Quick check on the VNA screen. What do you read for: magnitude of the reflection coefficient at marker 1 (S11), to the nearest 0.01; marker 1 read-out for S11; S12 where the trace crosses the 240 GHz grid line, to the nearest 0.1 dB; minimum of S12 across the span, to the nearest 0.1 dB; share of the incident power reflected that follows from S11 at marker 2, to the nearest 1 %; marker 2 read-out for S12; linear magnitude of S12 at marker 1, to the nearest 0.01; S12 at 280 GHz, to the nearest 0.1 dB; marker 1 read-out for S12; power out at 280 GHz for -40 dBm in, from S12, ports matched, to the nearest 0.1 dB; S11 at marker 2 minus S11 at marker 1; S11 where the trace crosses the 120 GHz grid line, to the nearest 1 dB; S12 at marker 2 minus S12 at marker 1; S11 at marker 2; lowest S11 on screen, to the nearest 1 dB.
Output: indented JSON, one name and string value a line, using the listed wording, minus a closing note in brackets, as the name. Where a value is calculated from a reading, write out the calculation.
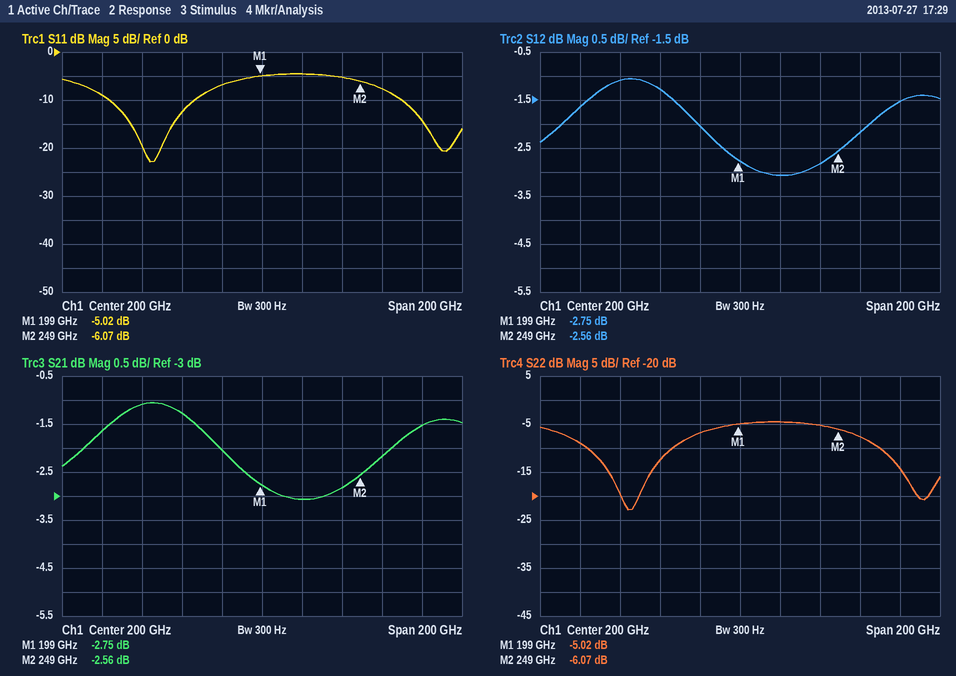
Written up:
{
  "magnitude of the reflection coefficient at marker 1 (S11), to the nearest 0.01": "10^(-5.02/20) ≈ 0.56",
  "marker 1 read-out for S11": "-5.02 dB",
  "S12 where the trace crosses the 240 GHz grid line, to the nearest 0.1 dB": "-2.8 dB",
  "minimum of S12 across the span, to the nearest 0.1 dB": "-3.1 dB",
  "share of the incident power reflected that follows from S11 at marker 2, to the nearest 1 %": "10^(-6.07/10) ≈ 25 %",
  "marker 2 read-out for S12": "-2.56 dB",
  "linear magnitude of S12 at marker 1, to the nearest 0.01": "10^(-2.75/20) ≈ 0.73",
  "S12 at 280 GHz, to the nearest 0.1 dB": "-1.5 dB",
  "marker 1 read-out for S12": "-2.75 dB",
  "power out at 280 GHz for -40 dBm in, from S12, ports matched, to the nearest 0.1 dB": "-40 dBm + (-1.5 dB) = -41.5 dBm",
  "S11 at marker 2 minus S11 at marker 1": "-6.07 − (-5.02) = -1.05 dB",
  "S11 where the trace crosses the 120 GHz grid line, to the nearest 1 dB": "-9 dB",
  "S12 at marker 2 minus S12 at marker 1": "-2.56 − (-2.75) = 0.19 dB",
  "S11 at marker 2": "-6.07 dB",
  "lowest S11 on screen, to the nearest 1 dB": "-23 dB"
}
